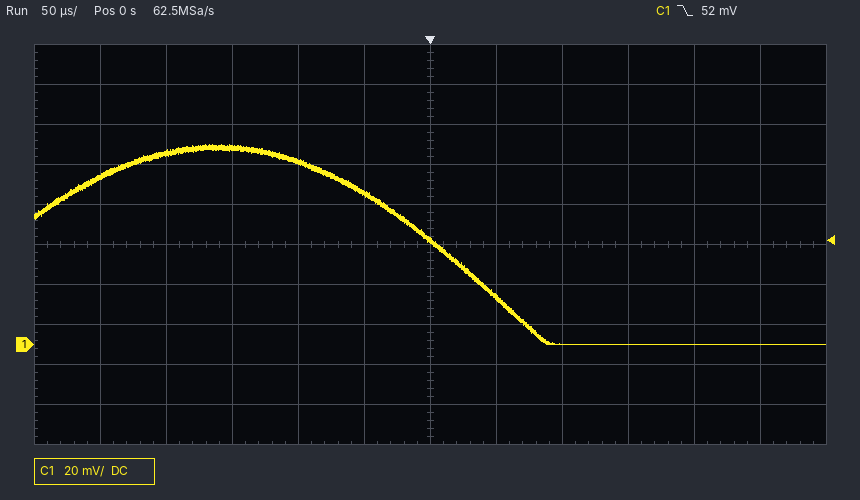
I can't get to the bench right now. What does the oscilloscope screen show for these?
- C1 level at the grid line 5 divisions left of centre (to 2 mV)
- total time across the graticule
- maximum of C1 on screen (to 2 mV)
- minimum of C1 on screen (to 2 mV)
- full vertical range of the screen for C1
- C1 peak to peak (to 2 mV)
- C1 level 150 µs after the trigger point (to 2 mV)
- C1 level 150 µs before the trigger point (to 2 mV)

84 mV
600 µs
100 mV
0 mV
200 mV
100 mV
0 mV
98 mV
